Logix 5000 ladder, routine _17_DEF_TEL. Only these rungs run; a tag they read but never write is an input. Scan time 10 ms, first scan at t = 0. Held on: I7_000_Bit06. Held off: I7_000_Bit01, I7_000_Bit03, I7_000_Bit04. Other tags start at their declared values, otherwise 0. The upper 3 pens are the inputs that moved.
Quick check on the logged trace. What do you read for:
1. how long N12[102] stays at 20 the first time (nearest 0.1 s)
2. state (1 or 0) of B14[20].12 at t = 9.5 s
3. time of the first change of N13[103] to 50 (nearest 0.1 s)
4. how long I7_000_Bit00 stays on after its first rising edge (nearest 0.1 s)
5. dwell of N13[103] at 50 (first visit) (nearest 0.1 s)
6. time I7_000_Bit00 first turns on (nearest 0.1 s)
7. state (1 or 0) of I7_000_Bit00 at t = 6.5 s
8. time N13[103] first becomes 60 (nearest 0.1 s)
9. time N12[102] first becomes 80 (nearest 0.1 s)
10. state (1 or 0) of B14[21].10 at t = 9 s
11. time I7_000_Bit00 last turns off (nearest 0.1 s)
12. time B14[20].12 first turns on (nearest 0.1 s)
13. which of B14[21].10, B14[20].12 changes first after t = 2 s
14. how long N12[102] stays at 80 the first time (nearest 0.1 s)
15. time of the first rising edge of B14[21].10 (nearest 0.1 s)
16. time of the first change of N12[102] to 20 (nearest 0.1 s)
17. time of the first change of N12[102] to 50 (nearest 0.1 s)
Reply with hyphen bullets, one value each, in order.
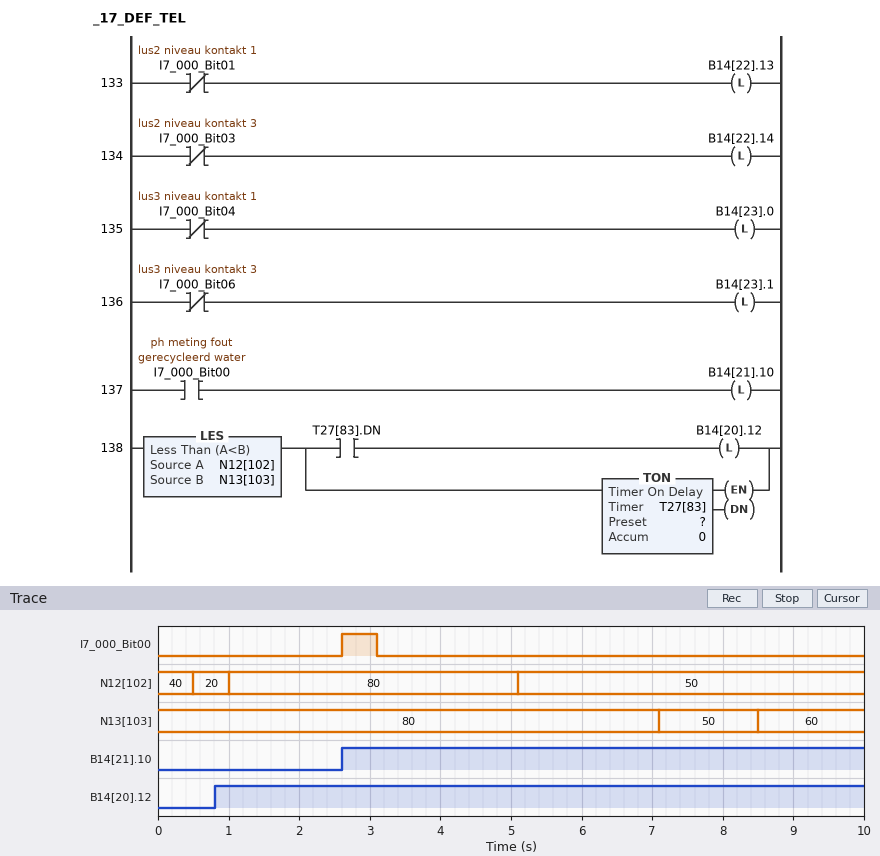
- 0.5 s
- 1
- 7.1 s
- 0.5 s
- 1.4 s
- 2.6 s
- 0
- 8.5 s
- 1.0 s
- 1
- 3.1 s
- 0.8 s
- B14[21].10
- 4.1 s
- 2.6 s
- 0.5 s
- 5.1 s
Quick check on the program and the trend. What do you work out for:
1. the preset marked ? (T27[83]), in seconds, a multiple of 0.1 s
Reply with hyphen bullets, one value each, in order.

- 0.8 s
